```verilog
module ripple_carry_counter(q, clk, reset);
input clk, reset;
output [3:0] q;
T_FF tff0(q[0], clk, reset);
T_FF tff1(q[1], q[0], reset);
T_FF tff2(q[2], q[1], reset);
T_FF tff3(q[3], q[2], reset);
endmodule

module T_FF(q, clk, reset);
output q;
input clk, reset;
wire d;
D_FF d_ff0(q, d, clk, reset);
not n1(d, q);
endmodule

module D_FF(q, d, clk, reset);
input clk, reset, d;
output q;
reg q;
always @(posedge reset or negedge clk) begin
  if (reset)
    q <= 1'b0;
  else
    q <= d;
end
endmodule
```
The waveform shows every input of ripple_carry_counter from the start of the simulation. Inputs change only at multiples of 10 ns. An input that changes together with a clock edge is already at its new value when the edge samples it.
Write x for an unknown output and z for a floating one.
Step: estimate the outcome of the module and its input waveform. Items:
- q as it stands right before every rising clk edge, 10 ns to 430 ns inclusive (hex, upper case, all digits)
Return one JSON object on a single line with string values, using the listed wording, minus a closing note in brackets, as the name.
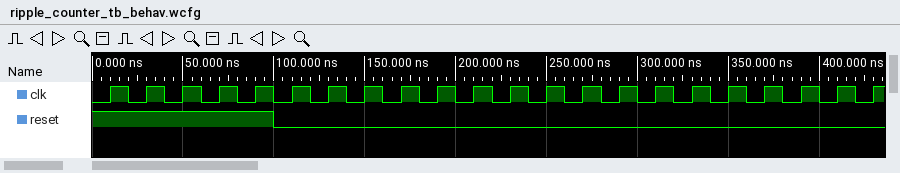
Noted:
{"q as it stands right before every rising clk edge, 10 ns to 430 ns inclusive": "0, 0, 0, 0, 0, 1, 2, 3, 4, 5, 6, 7, 8, 9, A, B, C, D, E, F, 0, 1"}
